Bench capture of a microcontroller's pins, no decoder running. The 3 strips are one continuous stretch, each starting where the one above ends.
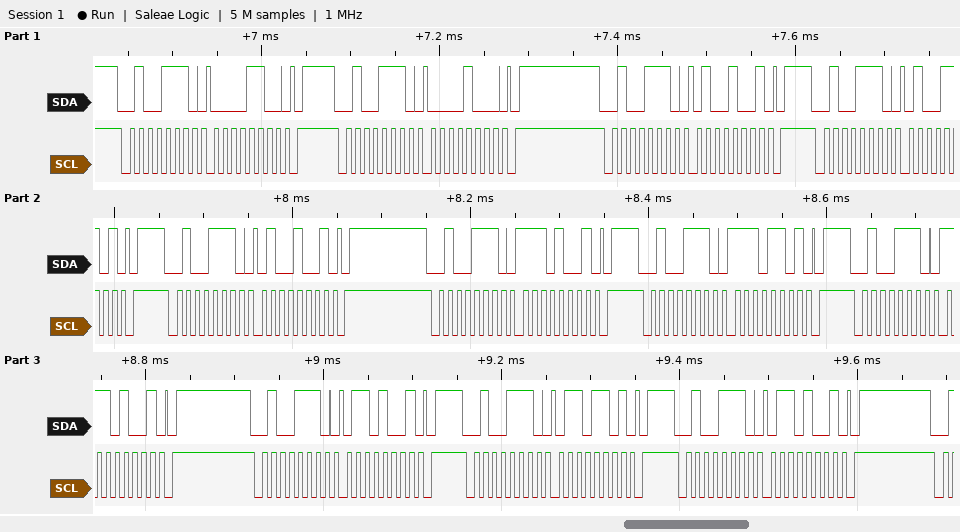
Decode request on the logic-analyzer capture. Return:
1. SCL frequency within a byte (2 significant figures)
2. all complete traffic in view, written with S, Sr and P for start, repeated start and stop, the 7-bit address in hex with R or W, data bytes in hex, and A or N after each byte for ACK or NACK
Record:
100 kHz
S 27W A 0C A P S 27W A 08 A P S 27W A 49 A P S 27W A 4D A P S 27W A 49 A P S 27W A E9 A P S 27W A ED A P S 27W A E9 A P S 27W A 69 A P S 27W A 6D A P S 27W A 69 A P
